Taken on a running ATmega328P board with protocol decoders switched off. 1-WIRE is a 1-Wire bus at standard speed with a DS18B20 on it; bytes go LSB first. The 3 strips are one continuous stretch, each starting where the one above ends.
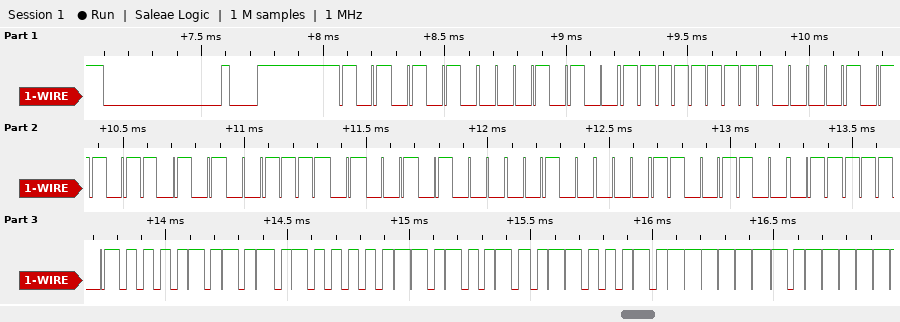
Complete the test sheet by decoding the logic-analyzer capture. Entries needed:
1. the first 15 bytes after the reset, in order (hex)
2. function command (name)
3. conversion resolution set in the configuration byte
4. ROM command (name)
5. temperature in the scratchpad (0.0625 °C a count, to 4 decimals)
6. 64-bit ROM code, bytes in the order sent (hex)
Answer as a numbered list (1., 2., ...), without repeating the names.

1. 55 28 FF A1 AD BC 14 04 33 BE 50 05 4B 46 7F
2. Read Scratchpad
3. 12 bits
4. Match ROM
5. 85.0000 °C
6. 28 FF A1 AD BC 14 04 33
